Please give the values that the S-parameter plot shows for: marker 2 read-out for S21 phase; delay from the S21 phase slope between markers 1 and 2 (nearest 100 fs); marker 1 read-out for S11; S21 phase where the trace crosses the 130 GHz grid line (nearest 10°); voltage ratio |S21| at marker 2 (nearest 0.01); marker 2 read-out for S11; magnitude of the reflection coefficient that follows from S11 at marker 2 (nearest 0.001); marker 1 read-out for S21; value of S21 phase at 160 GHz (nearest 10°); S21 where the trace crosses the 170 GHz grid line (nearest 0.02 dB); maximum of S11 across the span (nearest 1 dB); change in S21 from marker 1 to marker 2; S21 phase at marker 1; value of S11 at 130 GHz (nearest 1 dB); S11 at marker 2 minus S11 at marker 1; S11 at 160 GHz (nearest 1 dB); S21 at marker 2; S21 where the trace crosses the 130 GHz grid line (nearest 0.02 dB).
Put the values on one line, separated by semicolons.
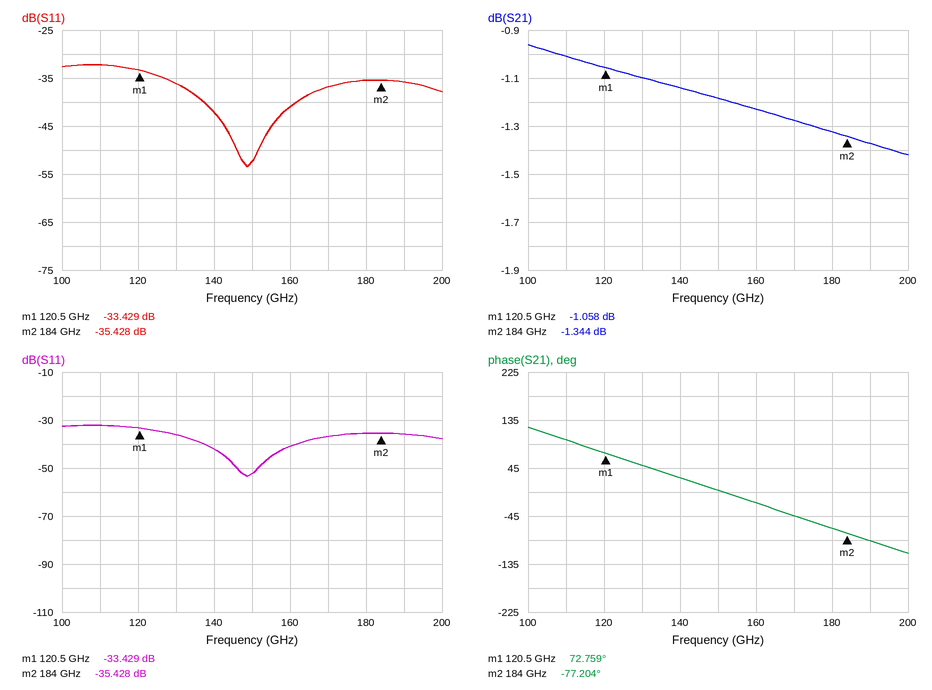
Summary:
-77.204°; 6.6 ps; -33.429 dB; 50°; 0.86; -35.428 dB; 0.017; -1.058 dB; -20°; -1.28 dB; -32 dB; -0.286 dB; 72.759°; -36 dB; -1.999 dB; -41 dB; -1.344 dB; -1.10 dB
